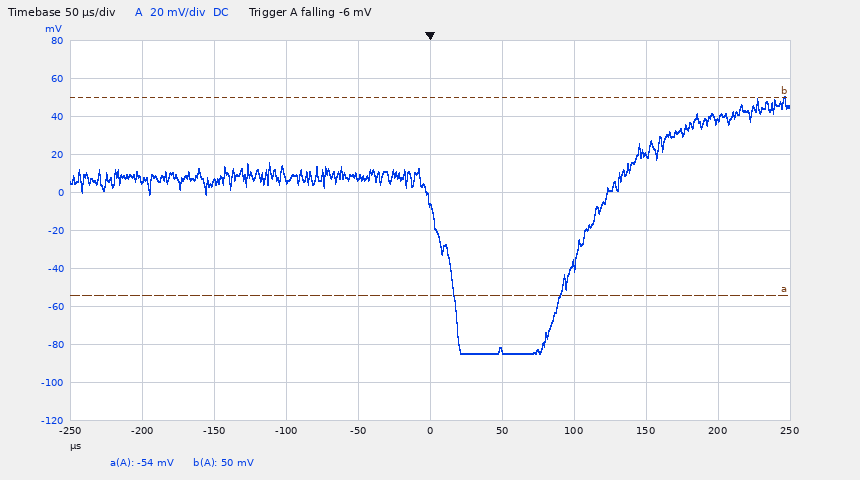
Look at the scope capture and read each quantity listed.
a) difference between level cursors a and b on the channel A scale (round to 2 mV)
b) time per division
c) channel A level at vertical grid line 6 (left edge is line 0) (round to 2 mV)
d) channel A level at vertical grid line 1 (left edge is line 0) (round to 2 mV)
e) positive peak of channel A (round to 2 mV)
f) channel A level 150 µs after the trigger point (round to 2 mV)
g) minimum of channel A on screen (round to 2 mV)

104 mV
50 µs
-84 mV
6 mV
50 mV
20 mV
-84 mV
